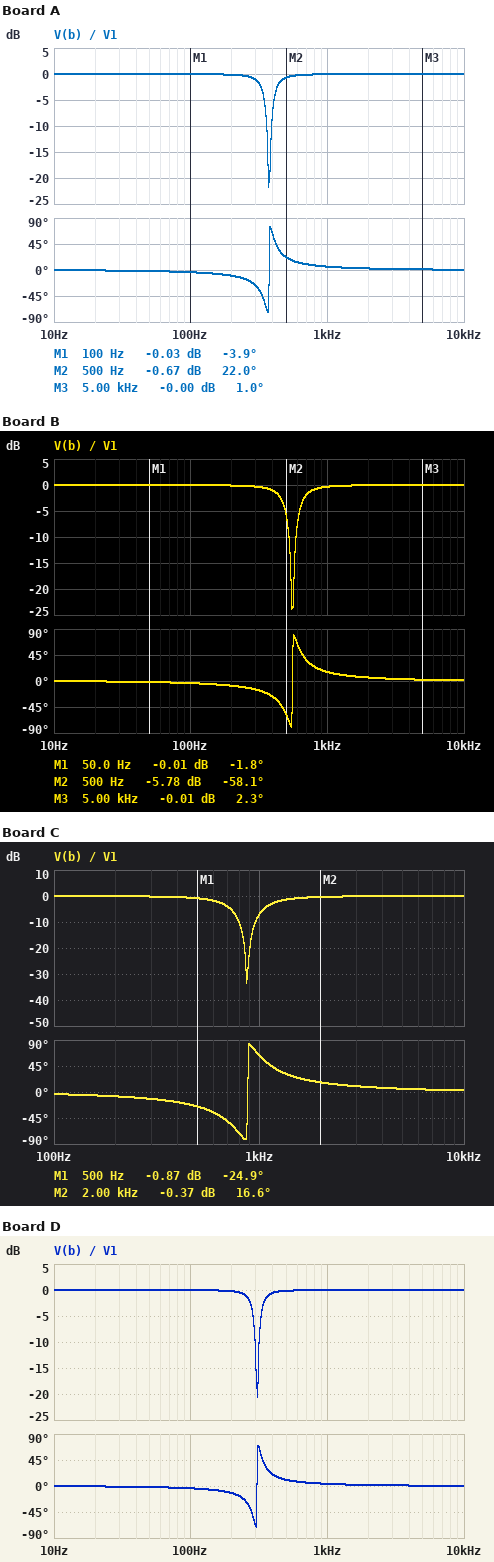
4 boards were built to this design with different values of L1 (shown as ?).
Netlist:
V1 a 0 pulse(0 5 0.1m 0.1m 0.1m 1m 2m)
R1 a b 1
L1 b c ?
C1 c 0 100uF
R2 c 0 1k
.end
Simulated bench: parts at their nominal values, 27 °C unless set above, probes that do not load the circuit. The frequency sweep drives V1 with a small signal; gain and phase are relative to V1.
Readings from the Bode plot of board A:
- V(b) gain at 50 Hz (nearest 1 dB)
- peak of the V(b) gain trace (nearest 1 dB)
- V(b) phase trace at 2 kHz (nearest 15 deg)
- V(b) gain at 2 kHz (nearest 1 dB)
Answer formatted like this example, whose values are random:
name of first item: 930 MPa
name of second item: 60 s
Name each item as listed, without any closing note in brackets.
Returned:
V(b) gain at 50 Hz: 0 dB
peak of the V(b) gain trace: 0 dB
V(b) phase trace at 2 kHz: 0 deg
V(b) gain at 2 kHz: 0 dB
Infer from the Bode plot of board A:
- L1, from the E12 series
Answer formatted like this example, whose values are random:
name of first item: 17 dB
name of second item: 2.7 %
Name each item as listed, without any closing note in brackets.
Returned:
L1, from the E12 series: 1.8 mH
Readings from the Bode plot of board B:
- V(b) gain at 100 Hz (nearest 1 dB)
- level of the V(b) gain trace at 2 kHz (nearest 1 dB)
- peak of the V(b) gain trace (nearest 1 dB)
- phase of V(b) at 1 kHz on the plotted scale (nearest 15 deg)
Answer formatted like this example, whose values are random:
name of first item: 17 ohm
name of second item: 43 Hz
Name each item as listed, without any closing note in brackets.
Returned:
V(b) gain at 100 Hz: 0 dB
level of the V(b) gain trace at 2 kHz: 0 dB
peak of the V(b) gain trace: 0 dB
phase of V(b) at 1 kHz on the plotted scale: 15 deg
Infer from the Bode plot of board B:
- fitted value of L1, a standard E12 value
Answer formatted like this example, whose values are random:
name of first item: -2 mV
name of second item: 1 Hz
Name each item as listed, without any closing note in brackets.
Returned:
fitted value of L1, a standard E12 value: 820 µH
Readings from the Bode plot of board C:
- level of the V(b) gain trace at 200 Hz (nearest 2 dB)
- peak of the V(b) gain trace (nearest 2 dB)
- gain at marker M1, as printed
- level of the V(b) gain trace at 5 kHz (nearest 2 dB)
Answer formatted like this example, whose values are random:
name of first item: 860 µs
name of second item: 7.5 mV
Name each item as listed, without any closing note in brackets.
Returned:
level of the V(b) gain trace at 200 Hz: 0 dB
peak of the V(b) gain trace: 0 dB
gain at marker M1, as printed: -0.87 dB
level of the V(b) gain trace at 5 kHz: 0 dB
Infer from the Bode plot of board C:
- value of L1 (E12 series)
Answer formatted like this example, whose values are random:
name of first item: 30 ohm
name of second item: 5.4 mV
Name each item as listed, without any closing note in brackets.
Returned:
value of L1: 330 µH
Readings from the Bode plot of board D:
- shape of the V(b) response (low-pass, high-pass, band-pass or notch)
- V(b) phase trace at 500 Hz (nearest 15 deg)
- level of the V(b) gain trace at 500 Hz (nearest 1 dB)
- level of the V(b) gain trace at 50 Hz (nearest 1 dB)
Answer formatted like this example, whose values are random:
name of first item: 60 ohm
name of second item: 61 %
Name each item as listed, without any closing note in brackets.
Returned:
shape of the V(b) response: notch
V(b) phase trace at 500 Hz: 15 deg
level of the V(b) gain trace at 500 Hz: 0 dB
level of the V(b) gain trace at 50 Hz: 0 dB
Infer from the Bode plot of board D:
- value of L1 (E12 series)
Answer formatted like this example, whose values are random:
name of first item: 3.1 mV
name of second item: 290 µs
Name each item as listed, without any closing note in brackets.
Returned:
value of L1: 2.7 mH
